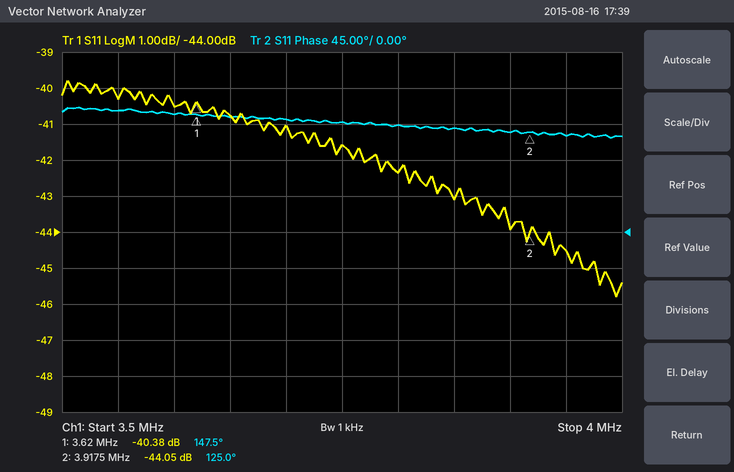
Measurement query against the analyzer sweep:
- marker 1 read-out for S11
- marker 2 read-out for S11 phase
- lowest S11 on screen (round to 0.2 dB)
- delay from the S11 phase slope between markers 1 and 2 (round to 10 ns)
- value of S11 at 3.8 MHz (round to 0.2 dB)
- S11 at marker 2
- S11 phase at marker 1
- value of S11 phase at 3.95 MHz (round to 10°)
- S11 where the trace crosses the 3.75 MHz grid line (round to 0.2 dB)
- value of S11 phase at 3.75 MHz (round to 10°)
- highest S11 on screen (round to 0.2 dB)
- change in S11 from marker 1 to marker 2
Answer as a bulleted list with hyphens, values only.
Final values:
- -40.38 dB
- 125.0°
- -45.8 dB
- 210 ns
- -42.4 dB
- -44.05 dB
- 147.5°
- 120°
- -41.6 dB
- 140°
- -39.8 dB
- -3.67 dB
